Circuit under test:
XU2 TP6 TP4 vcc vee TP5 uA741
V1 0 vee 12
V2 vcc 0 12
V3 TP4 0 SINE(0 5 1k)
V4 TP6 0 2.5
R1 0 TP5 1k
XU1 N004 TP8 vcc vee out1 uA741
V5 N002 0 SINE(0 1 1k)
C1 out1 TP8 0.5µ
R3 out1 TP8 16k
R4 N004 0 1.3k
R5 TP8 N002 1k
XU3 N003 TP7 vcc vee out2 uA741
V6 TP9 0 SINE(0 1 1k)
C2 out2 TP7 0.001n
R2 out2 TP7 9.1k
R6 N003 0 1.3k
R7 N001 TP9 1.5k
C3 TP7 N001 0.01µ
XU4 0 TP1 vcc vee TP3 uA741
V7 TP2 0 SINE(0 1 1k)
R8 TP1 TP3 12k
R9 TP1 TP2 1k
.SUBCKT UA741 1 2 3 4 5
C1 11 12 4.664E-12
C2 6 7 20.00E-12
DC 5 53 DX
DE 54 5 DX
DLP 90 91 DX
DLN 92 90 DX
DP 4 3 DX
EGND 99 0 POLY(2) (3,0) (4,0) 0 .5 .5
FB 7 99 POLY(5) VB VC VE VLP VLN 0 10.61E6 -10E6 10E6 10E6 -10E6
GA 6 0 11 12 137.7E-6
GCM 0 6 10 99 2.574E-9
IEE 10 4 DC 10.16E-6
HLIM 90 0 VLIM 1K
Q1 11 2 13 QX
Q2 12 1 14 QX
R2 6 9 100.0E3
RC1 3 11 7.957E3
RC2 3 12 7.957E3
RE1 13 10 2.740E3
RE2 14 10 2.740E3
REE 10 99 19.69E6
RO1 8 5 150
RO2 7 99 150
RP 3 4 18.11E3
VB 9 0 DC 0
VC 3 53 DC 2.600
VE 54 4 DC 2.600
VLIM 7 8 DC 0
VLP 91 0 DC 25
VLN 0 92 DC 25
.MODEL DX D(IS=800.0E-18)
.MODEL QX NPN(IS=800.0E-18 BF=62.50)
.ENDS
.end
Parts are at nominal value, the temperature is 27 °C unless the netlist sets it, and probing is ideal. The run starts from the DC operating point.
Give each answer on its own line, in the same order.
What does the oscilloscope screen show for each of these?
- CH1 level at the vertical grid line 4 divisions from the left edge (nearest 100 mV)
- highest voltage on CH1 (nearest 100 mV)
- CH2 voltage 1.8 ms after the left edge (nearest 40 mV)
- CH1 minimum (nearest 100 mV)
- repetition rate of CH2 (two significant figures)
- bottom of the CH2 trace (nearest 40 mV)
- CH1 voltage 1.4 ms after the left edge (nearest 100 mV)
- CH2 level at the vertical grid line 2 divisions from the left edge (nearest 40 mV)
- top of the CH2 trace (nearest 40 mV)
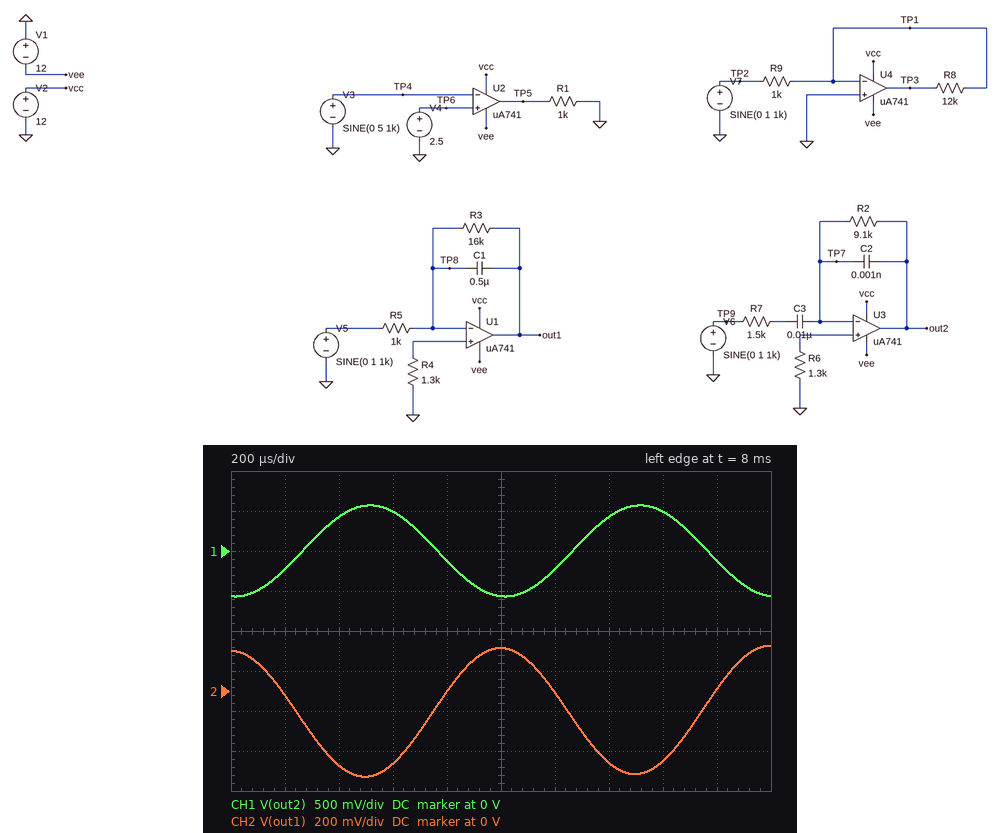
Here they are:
-100 mV
600 mV
0 V
-600 mV
1.0 kHz
-440 mV
400 mV
-360 mV
240 mV
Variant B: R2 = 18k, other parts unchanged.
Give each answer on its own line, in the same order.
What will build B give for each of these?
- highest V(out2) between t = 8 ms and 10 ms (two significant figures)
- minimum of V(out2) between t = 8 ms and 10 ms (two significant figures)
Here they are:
1.1 V
-1.1 V
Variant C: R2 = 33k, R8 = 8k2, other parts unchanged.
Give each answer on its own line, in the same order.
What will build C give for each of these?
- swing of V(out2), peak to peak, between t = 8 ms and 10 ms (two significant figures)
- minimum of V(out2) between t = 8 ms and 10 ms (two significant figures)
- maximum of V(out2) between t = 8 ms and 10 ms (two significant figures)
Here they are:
4.1 V
-2.1 V
2.1 V
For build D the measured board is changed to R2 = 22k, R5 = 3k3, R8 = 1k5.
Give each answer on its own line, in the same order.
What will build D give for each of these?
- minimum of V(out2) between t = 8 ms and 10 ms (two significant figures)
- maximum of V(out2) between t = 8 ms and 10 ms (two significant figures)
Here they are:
-1.4 V
1.4 V
